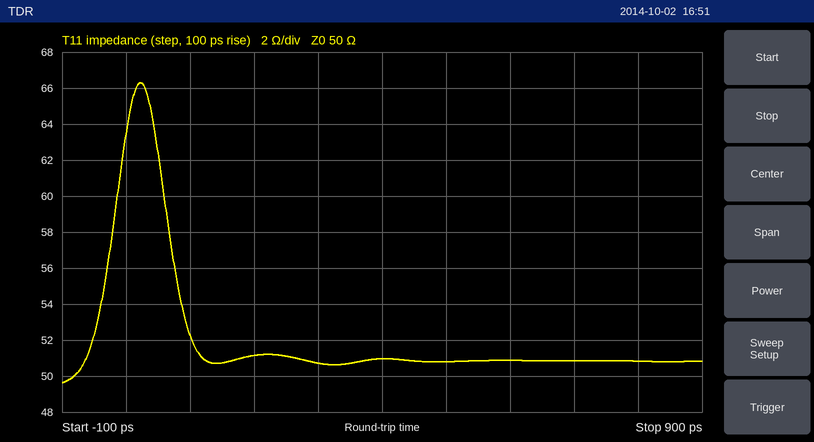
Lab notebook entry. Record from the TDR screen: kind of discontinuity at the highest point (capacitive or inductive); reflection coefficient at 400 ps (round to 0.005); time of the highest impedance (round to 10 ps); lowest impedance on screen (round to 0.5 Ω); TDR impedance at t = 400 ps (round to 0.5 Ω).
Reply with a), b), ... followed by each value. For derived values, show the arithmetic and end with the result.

a) inductive
b) (51 − 50)/(51 + 50) ≈ +0.010
c) 20 ps
d) 49.5 Ω
e) 51.0 Ω
